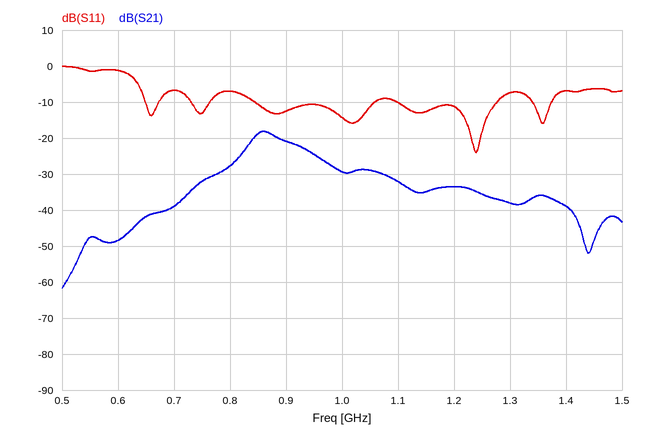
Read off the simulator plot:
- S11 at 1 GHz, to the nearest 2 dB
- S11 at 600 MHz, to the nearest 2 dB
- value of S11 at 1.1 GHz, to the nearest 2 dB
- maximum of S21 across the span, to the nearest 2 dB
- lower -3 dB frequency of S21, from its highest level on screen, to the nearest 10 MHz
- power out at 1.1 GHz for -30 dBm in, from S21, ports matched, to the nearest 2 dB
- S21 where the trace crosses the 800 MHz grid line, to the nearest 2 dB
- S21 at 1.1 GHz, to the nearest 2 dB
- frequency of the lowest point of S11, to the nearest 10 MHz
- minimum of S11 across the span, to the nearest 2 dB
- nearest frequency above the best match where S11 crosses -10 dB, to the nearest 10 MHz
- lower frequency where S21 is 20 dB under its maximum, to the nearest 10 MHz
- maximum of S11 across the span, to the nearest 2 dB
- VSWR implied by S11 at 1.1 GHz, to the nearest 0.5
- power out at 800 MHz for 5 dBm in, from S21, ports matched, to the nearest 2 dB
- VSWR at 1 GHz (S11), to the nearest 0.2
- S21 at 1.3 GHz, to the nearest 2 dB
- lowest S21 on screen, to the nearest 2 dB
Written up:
-14 dB
-2 dB
-10 dB
-18 dB
840 MHz
-62 dBm
-28 dB
-32 dB
1.24 GHz
-24 dB
1.28 GHz
710 MHz
0 dB
2.0
-22 dBm
1.4
-38 dB
-62 dB
